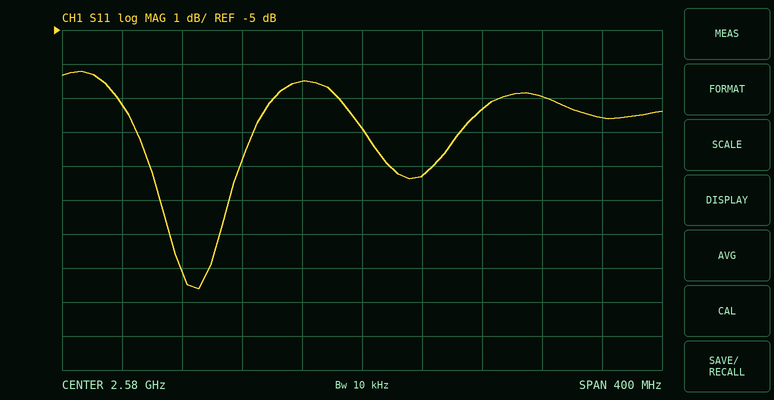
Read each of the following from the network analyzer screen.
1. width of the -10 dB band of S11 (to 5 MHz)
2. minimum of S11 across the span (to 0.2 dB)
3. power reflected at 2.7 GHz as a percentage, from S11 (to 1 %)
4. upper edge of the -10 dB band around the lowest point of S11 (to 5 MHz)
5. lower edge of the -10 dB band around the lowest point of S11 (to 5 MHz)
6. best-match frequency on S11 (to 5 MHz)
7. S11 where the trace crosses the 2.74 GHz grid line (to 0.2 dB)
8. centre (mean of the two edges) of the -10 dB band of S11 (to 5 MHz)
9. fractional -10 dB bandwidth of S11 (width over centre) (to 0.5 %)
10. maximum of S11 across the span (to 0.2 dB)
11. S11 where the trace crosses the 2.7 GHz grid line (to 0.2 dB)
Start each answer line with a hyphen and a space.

- 45 MHz
- -12.6 dB
- 20 %
- 2.490 GHz
- 2.445 GHz
- 2.470 GHz
- -7.6 dB
- 2.470 GHz
- 2.0 %
- -6.2 dB
- -7.0 dB
